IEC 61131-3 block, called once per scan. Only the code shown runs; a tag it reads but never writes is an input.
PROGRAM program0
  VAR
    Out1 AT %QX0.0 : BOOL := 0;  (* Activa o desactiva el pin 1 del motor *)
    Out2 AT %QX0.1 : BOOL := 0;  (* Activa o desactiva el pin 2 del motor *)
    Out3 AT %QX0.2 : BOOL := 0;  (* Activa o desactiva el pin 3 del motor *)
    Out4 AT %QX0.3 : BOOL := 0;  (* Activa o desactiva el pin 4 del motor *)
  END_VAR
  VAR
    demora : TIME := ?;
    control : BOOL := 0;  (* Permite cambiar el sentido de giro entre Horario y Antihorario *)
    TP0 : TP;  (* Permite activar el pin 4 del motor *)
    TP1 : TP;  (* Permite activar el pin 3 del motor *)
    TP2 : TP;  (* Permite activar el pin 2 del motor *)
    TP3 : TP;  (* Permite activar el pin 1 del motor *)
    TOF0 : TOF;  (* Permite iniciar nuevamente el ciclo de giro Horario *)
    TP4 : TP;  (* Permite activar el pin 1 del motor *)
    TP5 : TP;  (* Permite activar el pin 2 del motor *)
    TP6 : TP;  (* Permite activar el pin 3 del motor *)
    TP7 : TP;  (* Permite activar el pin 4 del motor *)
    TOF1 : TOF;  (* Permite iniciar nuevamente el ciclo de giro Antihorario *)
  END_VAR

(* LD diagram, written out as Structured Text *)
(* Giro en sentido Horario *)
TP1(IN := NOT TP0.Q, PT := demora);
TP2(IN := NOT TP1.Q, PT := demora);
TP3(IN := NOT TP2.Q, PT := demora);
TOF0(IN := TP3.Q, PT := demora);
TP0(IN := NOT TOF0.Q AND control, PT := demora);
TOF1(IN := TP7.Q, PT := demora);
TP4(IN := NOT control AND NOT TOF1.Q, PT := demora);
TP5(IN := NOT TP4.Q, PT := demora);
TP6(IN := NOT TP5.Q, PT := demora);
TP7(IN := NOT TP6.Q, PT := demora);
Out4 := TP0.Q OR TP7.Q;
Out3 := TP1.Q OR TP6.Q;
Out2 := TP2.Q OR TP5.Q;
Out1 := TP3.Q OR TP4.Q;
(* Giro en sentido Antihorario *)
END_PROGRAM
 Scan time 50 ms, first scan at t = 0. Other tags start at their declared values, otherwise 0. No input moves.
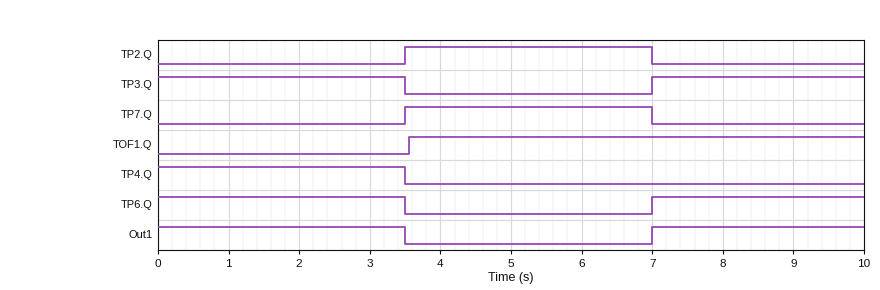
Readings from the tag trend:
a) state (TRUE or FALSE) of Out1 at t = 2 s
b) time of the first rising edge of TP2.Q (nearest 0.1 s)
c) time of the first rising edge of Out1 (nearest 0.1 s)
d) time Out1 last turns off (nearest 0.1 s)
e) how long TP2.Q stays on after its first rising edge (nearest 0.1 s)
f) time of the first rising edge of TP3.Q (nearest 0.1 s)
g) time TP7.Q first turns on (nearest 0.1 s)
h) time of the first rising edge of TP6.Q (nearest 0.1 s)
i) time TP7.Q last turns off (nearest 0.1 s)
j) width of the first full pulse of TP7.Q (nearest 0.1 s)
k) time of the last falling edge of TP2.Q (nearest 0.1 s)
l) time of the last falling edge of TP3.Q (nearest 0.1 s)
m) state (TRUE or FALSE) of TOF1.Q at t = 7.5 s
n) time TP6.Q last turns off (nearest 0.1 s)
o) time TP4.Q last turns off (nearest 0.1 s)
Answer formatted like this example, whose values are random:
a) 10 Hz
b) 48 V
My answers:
a) TRUE
b) 3.5 s
c) 7.0 s
d) 3.5 s
e) 3.5 s
f) 7.0 s
g) 3.5 s
h) 7.0 s
i) 7.0 s
j) 3.5 s
k) 7.0 s
l) 3.5 s
m) TRUE
n) 3.5 s
o) 3.5 s
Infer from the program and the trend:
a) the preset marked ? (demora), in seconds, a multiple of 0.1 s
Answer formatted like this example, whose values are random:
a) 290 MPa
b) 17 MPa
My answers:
a) 3.5 s
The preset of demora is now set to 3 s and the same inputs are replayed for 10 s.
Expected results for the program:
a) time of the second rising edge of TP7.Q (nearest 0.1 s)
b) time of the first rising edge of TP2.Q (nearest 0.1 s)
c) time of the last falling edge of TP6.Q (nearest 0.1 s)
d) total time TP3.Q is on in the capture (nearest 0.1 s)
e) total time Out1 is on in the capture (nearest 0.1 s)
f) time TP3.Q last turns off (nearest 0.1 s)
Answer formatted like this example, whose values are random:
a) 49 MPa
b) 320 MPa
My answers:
a) 9.0 s
b) 3.0 s
c) 9.0 s
d) 6.0 s
e) 6.0 s
f) 9.0 s
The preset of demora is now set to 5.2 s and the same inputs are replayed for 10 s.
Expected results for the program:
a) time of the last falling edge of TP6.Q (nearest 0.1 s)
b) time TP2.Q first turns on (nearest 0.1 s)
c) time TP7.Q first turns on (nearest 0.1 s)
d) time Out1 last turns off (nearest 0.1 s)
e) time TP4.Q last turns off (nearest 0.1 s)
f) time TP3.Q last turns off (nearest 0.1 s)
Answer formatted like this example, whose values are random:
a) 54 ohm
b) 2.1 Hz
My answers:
a) 5.2 s
b) 5.2 s
c) 5.2 s
d) 5.2 s
e) 5.2 s
f) 5.2 s
